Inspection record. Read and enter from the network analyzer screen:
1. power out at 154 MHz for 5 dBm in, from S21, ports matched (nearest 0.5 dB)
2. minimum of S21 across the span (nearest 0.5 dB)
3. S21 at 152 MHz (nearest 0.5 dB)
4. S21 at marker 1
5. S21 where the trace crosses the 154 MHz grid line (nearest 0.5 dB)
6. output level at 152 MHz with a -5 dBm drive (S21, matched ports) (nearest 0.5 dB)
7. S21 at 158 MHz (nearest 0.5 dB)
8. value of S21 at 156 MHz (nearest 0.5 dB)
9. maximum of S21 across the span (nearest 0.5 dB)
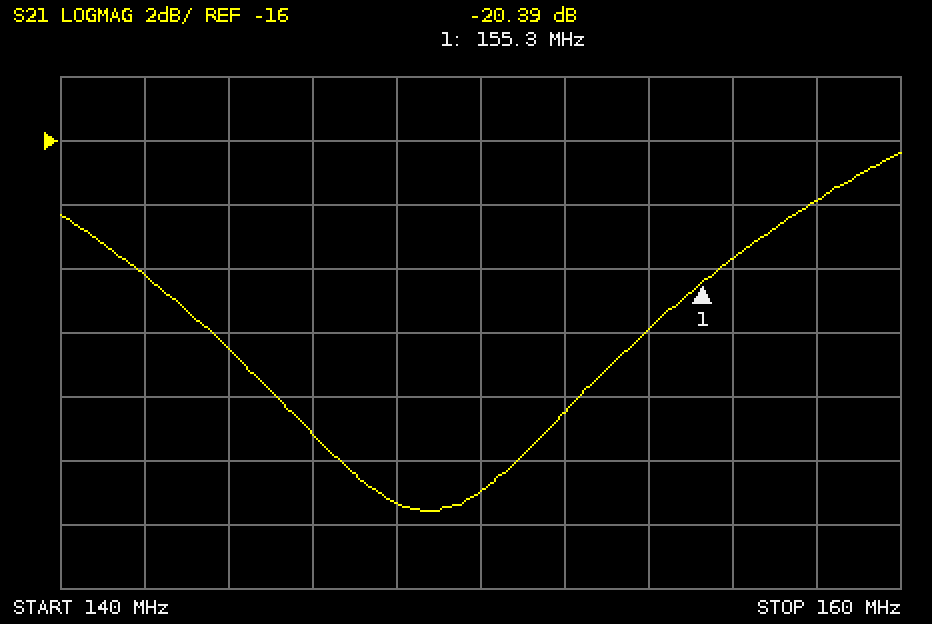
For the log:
-17.0 dBm
-27.5 dB
-24.5 dB
-20.39 dB
-22.0 dB
-29.5 dBm
-18.0 dB
-19.5 dB
-16.5 dB
